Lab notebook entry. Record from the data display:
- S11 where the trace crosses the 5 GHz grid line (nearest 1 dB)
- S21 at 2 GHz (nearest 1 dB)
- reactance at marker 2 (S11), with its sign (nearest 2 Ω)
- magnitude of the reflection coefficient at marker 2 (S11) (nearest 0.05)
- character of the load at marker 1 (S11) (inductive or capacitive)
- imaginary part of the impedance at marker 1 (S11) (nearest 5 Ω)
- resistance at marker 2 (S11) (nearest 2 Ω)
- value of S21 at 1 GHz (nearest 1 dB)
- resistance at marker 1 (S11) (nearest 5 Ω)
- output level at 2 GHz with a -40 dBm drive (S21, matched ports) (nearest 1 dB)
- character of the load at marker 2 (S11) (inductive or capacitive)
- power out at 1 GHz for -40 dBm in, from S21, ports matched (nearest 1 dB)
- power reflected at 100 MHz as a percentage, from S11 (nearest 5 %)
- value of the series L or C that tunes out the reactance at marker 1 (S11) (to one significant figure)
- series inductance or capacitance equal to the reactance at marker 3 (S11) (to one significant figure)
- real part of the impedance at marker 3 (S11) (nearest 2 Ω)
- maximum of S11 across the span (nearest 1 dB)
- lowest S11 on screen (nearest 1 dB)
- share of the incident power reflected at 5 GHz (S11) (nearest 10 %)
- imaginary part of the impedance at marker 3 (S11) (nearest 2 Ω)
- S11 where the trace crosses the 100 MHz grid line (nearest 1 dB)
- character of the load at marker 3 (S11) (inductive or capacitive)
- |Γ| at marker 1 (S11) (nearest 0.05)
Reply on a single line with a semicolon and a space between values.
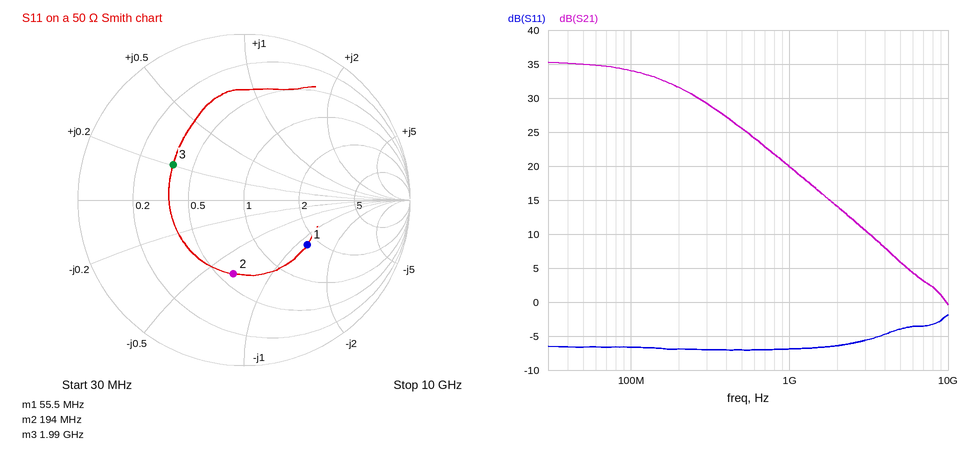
-4 dB; 14 dB; -34 Ω; 0.45; capacitive; -60 Ω; 30 Ω; 20 dB; 85 Ω; -26 dBm; capacitive; -20 dBm; 20 %; 200 nH; 800 pH; 18 Ω; -2 dB; -7 dB; 40 %; +10 Ω; -7 dB; inductive; 0.45
